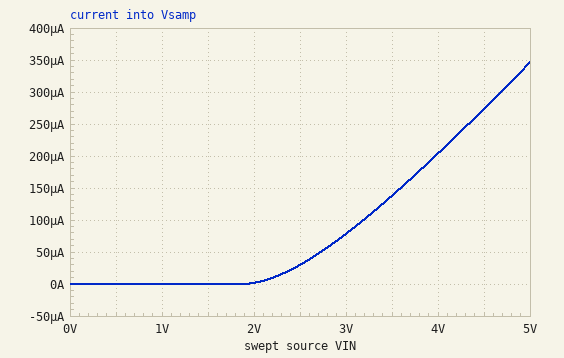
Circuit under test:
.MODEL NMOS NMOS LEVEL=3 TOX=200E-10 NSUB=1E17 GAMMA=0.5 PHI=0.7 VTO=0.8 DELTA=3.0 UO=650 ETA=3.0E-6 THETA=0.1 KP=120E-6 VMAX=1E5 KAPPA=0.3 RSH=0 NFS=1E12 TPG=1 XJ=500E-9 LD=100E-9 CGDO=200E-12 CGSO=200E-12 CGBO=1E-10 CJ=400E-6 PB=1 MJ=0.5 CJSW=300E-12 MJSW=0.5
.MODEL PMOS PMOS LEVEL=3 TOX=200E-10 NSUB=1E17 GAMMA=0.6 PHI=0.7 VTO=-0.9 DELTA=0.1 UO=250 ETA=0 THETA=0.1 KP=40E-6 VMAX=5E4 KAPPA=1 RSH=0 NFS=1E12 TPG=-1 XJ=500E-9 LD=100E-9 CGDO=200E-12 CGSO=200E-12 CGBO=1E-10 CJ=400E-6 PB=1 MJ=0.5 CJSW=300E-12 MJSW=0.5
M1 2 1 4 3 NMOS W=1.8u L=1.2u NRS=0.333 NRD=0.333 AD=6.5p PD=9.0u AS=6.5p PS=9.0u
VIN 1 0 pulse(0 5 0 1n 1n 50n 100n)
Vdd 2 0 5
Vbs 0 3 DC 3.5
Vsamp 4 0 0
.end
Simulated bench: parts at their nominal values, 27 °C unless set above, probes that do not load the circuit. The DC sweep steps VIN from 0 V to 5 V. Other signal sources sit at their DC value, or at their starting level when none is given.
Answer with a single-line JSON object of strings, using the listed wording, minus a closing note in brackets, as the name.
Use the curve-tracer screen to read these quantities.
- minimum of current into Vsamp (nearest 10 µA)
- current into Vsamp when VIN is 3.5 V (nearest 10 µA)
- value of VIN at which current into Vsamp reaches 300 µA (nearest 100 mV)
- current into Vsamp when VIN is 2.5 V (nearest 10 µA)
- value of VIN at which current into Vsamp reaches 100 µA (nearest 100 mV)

{"minimum of current into Vsamp": "0 A", "current into Vsamp when VIN is 3.5 V": "140 µA", "value of VIN at which current into Vsamp reaches 300 µA": "4.7 V", "current into Vsamp when VIN is 2.5 V": "30 µA", "value of VIN at which current into Vsamp reaches 100 µA": "3.2 V"}
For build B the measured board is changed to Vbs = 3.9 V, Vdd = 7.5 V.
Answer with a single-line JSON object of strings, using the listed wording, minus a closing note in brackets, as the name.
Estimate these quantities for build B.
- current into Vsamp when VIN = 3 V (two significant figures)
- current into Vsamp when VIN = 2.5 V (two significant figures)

{"current into Vsamp when VIN = 3 V": "71 µA", "current into Vsamp when VIN = 2.5 V": "24 µA"}
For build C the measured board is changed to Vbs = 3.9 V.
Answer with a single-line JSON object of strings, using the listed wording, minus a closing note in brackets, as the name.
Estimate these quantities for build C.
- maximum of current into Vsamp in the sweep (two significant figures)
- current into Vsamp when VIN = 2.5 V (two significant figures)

{"maximum of current into Vsamp in the sweep": "330 µA", "current into Vsamp when VIN = 2.5 V": "23 µA"}
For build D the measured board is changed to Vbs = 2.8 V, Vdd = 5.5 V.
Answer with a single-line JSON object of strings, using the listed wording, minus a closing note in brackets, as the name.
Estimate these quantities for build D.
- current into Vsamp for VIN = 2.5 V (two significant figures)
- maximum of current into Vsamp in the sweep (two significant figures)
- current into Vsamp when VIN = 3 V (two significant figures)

{"current into Vsamp for VIN = 2.5 V": "45 µA", "maximum of current into Vsamp in the sweep": "370 µA", "current into Vsamp when VIN = 3 V": "98 µA"}
